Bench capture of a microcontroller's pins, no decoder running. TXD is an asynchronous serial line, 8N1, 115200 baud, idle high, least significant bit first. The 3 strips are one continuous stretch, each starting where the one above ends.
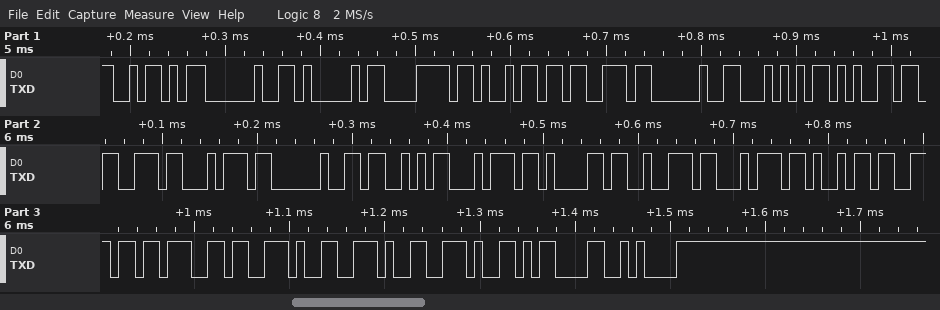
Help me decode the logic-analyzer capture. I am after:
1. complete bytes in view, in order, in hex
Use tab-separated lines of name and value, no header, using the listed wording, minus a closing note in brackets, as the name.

complete bytes in view, in order, in hex	0x5A 0x20 0x41 0x78 0x69 0x73 0x20 0x54 0x65 0x73 0x74 0x20 0x53 0x74 0x61 0x72 0x74 0x69 0x6E 0x67 0x2E 0x2E 0x2E 0x0D 0x0A
